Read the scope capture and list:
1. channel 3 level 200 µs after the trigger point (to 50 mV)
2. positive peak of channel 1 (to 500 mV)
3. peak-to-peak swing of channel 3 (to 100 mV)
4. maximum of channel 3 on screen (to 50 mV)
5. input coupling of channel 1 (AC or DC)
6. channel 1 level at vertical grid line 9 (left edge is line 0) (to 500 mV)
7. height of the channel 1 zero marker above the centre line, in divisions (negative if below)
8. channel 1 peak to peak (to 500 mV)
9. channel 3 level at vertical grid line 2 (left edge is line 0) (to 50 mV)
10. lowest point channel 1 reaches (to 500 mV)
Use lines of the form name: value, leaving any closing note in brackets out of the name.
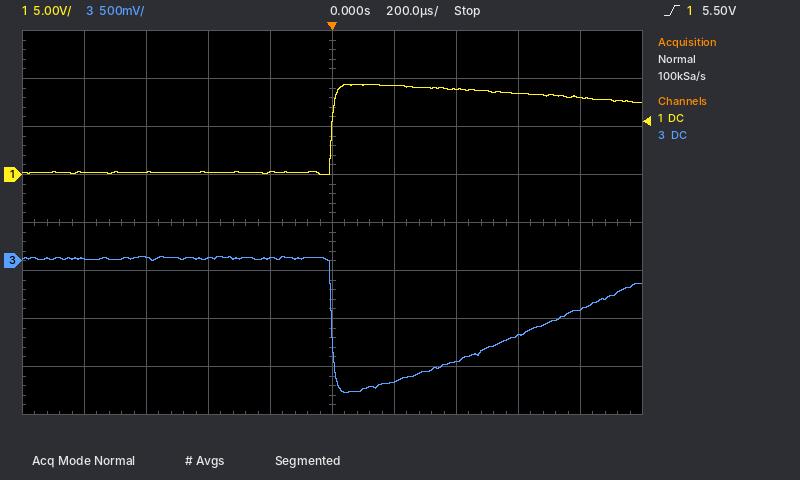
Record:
channel 3 level 200 µs after the trigger point: -1.25 V
positive peak of channel 1: 9.5 V
peak-to-peak swing of channel 3: 1.40 V
maximum of channel 3 on screen: 50 mV
input coupling of channel 1: DC
channel 1 level at vertical grid line 9 (left edge is line 0): 8.0 V
height of the channel 1 zero marker above the centre line, in divisions: +1.0 div
channel 1 peak to peak: 9.5 V
channel 3 level at vertical grid line 2 (left edge is line 0): 50 mV
lowest point channel 1 reaches: 0.0 V
